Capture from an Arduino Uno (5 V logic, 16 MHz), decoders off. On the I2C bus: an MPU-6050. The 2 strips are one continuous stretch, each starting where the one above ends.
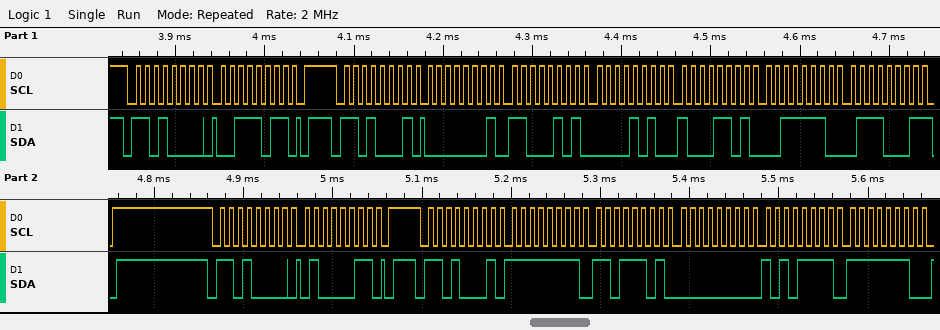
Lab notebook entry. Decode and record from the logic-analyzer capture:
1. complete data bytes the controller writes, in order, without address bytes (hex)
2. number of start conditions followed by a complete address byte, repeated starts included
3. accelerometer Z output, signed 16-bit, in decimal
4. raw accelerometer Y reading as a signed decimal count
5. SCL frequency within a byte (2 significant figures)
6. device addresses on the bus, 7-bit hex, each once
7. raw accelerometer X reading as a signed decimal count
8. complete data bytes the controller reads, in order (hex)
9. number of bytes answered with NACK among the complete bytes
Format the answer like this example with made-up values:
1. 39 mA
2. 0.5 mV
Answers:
1. 3B 43
2. 4
3. 15985
4. 2701
5. 100 kHz
6. 0x68
7. 453
8. 01 C5 0A 8D 3E 71 FF DD 00 AF FE
9. 1
